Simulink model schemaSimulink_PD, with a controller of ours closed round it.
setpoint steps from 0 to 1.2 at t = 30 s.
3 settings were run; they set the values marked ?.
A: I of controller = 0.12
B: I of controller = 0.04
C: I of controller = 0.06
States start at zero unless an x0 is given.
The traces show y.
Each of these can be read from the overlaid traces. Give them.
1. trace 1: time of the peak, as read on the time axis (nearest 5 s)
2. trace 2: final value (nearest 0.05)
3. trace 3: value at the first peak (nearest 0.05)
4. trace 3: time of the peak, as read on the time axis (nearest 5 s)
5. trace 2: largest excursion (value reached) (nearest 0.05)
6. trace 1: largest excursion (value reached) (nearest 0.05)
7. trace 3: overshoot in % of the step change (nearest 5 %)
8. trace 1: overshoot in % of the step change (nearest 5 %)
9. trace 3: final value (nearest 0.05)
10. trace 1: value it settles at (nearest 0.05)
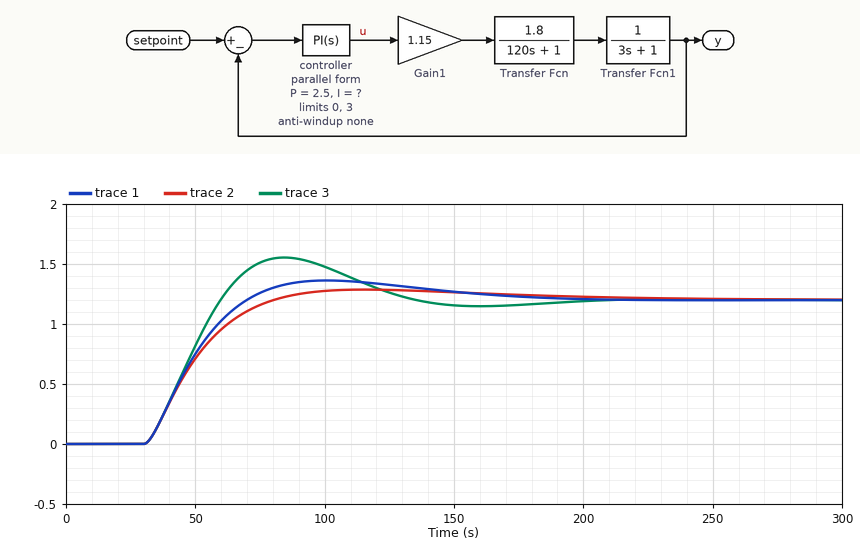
100 s
1.20
1.55
85 s
1.30
1.35
30 %
15 %
1.20
1.20
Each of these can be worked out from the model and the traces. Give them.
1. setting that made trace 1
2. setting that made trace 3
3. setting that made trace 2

C
A
B
